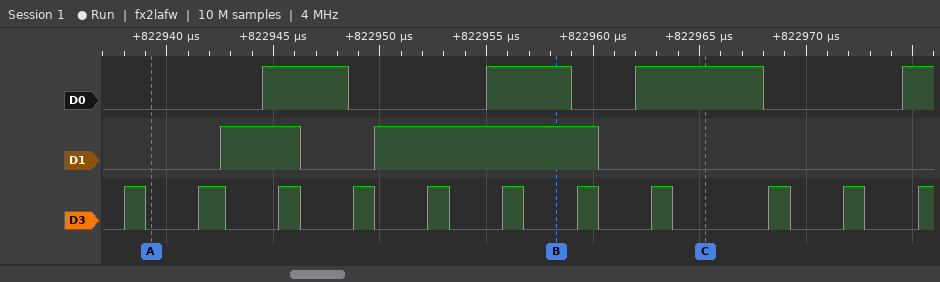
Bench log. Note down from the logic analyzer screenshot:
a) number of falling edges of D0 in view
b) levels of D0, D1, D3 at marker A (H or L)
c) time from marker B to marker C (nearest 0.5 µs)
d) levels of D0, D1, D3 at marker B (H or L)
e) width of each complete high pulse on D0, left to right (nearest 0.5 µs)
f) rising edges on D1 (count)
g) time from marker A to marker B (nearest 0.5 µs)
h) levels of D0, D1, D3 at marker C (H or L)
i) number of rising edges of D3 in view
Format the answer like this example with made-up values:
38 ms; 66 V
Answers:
3; D0=L, D1=L, D3=L; 7 µs; D0=H, D1=H, D3=L; 4 µs, 4 µs, 6 µs; 2; 19 µs; D0=H, D1=L, D3=L; 11
